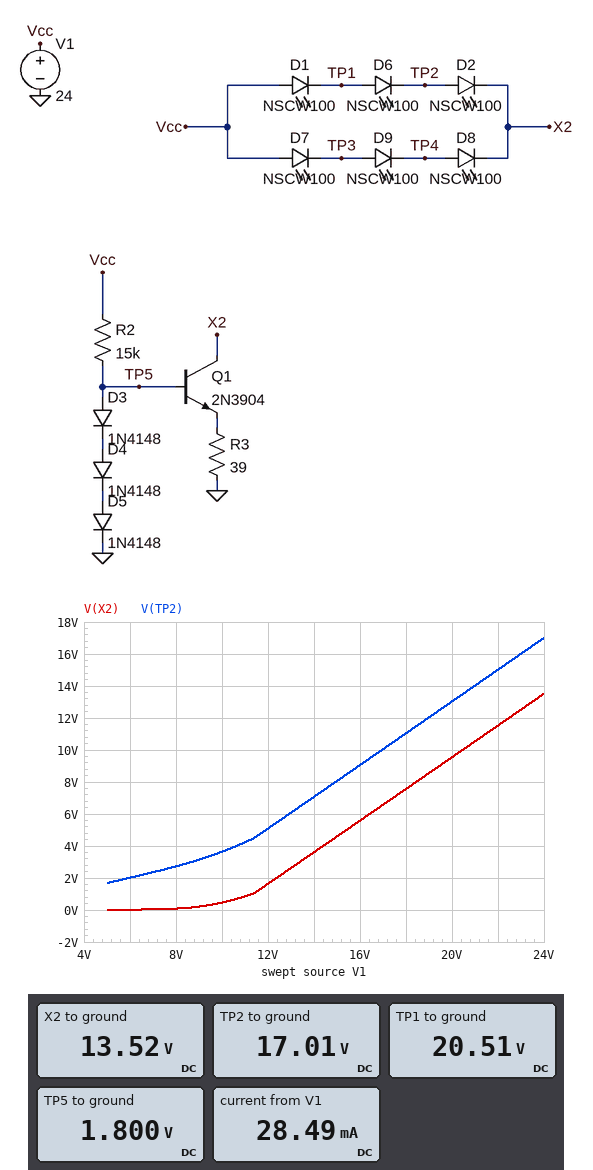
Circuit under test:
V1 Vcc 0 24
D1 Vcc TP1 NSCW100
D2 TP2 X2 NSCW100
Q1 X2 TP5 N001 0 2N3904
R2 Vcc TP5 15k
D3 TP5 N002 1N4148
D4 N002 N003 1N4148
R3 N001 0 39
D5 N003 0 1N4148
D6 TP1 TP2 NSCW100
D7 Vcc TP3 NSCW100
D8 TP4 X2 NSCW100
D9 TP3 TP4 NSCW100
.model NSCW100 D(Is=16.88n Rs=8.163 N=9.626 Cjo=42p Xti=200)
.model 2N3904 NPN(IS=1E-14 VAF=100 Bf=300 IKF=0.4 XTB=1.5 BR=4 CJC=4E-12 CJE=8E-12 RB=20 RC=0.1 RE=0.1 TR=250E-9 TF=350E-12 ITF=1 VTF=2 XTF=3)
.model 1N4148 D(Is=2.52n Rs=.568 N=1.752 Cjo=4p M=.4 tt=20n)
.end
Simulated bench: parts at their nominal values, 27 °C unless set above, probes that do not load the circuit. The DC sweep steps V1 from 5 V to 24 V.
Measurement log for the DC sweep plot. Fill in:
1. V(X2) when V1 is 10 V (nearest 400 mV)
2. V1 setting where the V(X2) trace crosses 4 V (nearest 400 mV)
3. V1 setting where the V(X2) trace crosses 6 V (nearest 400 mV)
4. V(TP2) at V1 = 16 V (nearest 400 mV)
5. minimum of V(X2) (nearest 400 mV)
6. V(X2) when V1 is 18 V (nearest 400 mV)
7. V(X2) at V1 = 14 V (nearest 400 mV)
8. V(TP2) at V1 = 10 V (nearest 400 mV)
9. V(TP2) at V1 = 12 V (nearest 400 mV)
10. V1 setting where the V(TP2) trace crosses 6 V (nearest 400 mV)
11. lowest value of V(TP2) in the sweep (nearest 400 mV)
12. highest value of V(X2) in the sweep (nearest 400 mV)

400 mV
14.4 V
16.4 V
9.2 V
0 V
7.6 V
3.6 V
3.6 V
5.2 V
12.8 V
1.6 V
13.6 V
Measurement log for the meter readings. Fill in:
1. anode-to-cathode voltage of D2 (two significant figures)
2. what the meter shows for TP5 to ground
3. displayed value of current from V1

3.5 V
1.800 V
28.49 mA
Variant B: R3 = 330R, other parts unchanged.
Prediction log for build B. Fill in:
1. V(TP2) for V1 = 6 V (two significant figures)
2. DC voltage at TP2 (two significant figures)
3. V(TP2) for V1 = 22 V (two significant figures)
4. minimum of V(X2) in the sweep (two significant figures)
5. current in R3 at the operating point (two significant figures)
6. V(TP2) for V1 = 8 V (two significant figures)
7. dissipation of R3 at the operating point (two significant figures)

2.1 V
18 V
16 V
110 mV
3.4 mA
3.0 V
3.8 mW
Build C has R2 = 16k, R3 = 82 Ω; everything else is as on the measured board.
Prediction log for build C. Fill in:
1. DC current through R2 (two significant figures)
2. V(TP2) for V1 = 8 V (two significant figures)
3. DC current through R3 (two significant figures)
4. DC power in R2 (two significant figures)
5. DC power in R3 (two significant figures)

1.4 mA
2.8 V
13 mA
31 mW
14 mW
